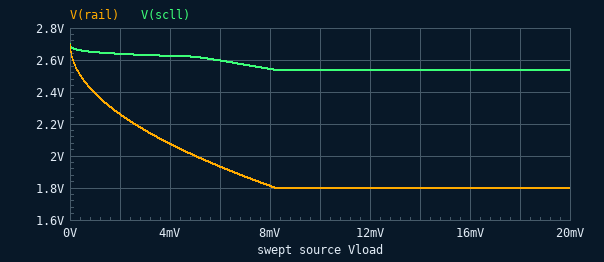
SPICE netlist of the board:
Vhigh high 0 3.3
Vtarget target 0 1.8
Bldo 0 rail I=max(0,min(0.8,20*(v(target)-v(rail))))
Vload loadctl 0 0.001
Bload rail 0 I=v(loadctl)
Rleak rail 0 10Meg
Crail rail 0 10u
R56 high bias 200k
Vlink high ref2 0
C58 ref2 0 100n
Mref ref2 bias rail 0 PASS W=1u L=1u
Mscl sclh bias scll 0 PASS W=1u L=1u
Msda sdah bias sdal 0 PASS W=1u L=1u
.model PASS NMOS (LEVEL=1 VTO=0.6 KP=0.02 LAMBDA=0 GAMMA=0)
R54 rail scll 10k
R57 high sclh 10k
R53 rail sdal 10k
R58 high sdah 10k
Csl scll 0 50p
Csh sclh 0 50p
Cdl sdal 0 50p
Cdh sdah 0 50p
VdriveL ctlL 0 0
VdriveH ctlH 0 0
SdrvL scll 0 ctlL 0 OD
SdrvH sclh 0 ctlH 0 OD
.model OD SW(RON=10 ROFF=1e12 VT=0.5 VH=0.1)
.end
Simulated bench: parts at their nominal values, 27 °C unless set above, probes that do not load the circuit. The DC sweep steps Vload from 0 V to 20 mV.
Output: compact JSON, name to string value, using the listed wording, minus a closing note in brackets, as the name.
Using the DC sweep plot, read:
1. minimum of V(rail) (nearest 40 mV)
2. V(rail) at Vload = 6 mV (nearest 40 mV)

{"minimum of V(rail)": "1.80 V", "V(rail) at Vload = 6 mV": "1.92 V"}
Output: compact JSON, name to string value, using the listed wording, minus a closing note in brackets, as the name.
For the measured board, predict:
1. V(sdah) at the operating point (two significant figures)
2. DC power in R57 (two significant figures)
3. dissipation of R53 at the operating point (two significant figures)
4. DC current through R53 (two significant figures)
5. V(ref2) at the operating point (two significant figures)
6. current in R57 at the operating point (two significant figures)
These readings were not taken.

{"V(sdah) at the operating point": "3.0 V", "DC power in R57": "6.6 µW", "dissipation of R53 at the operating point": "6.6 µW", "DC current through R53": "26 µA", "V(ref2) at the operating point": "3.3 V", "current in R57 at the operating point": "26 µA"}
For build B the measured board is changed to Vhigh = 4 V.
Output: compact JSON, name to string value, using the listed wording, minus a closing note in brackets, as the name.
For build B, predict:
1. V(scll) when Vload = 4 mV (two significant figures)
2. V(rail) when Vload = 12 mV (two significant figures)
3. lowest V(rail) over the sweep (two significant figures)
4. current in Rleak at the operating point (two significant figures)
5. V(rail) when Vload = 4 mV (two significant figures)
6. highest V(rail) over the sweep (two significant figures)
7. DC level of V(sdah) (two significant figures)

{"V(scll) when Vload = 4 mV": "3.3 V", "V(rail) when Vload = 12 mV": "2.3 V", "lowest V(rail) over the sweep": "2.0 V", "current in Rleak at the operating point": "310 nA", "V(rail) when Vload = 4 mV": "2.8 V", "highest V(rail) over the sweep": "3.4 V", "DC level of V(sdah)": "3.7 V"}
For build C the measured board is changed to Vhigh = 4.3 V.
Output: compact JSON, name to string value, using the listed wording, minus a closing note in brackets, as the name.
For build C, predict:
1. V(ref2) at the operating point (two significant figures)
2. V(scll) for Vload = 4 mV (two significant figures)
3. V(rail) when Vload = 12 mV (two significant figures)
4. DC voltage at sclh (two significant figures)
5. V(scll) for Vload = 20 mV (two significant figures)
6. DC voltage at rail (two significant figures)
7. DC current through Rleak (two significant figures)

{"V(ref2) at the operating point": "4.3 V", "V(scll) for Vload = 4 mV": "3.6 V", "V(rail) when Vload = 12 mV": "2.6 V", "DC voltage at sclh": "4.0 V", "V(scll) for Vload = 20 mV": "3.3 V", "DC voltage at rail": "3.4 V", "DC current through Rleak": "340 nA"}
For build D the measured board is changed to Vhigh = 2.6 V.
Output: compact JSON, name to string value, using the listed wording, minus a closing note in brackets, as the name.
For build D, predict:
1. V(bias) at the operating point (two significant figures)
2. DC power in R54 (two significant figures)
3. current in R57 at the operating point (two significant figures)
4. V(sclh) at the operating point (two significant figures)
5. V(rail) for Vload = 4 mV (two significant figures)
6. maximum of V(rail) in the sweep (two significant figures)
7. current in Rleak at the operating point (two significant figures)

{"V(bias) at the operating point": "2.6 V", "DC power in R54": "2.6 µW", "current in R57 at the operating point": "16 µA", "V(sclh) at the operating point": "2.4 V", "V(rail) for Vload = 4 mV": "1.8 V", "maximum of V(rail) in the sweep": "2.0 V", "current in Rleak at the operating point": "180 nA"}
